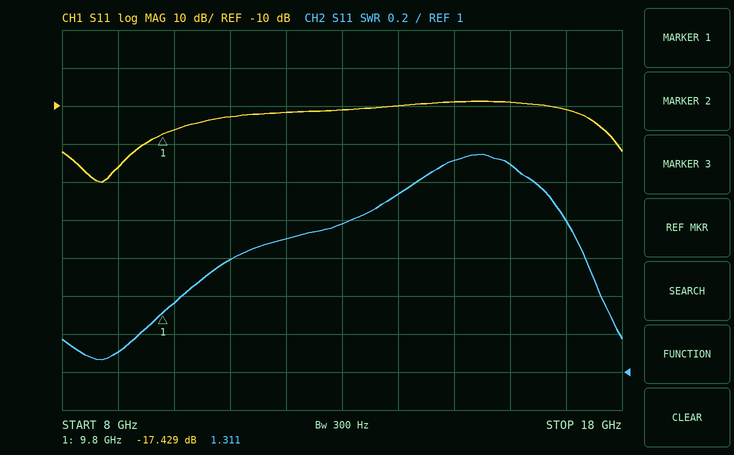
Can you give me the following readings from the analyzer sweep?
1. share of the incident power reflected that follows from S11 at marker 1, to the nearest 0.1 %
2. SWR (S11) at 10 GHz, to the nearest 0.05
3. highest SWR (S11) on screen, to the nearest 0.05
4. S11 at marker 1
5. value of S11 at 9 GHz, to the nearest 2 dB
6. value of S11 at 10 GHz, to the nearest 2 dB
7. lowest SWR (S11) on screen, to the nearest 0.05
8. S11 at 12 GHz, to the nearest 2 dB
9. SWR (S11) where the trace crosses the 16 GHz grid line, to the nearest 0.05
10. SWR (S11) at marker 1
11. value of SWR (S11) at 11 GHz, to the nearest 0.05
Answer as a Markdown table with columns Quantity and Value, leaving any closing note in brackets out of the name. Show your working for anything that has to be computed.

| Quantity | Value |
|---|---|
| share of the incident power reflected that follows from S11 at marker 1, to the nearest 0.1 % | 10^(-17.429/10) ≈ 1.8 % |
| SWR (S11) at 10 GHz, to the nearest 0.05 | 1.35 |
| highest SWR (S11) on screen, to the nearest 0.05 | 2.15 |
| S11 at marker 1 | -17.429 dB |
| value of S11 at 9 GHz, to the nearest 2 dB | -26 dB |
| value of S11 at 10 GHz, to the nearest 2 dB | -16 dB |
| lowest SWR (S11) on screen, to the nearest 0.05 | 1.05 |
| S11 at 12 GHz, to the nearest 2 dB | -12 dB |
| SWR (S11) where the trace crosses the 16 GHz grid line, to the nearest 0.05 | 2.10 |
| SWR (S11) at marker 1 | 1.311 |
| value of SWR (S11) at 11 GHz, to the nearest 0.05 | 1.60 |
